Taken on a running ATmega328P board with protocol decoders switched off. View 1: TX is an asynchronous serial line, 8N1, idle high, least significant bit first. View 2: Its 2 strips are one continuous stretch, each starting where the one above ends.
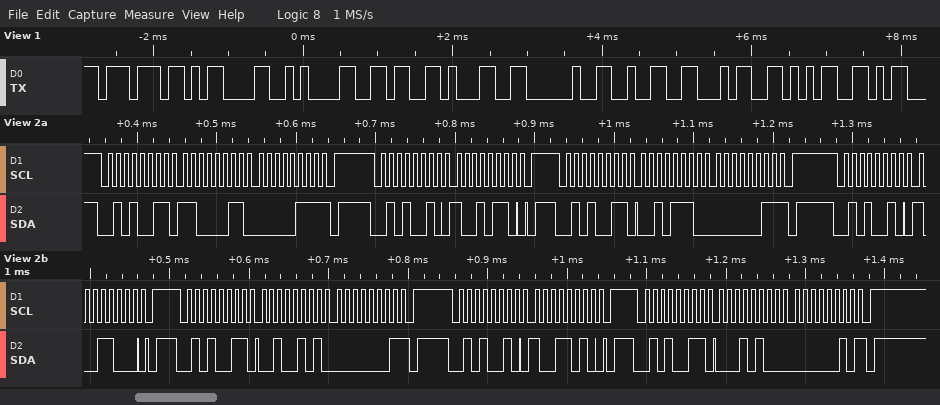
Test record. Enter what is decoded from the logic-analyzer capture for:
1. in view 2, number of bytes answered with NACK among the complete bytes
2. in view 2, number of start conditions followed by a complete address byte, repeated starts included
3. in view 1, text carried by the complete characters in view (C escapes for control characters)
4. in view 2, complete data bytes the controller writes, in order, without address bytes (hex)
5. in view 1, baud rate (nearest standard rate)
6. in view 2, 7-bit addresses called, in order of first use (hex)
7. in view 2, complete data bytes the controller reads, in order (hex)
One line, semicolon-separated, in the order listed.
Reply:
4; 7; "w\r\n61 245"; 96 98 9A; 9600 baud; 0x29; C3 07 2E 03 25 01 14 02
